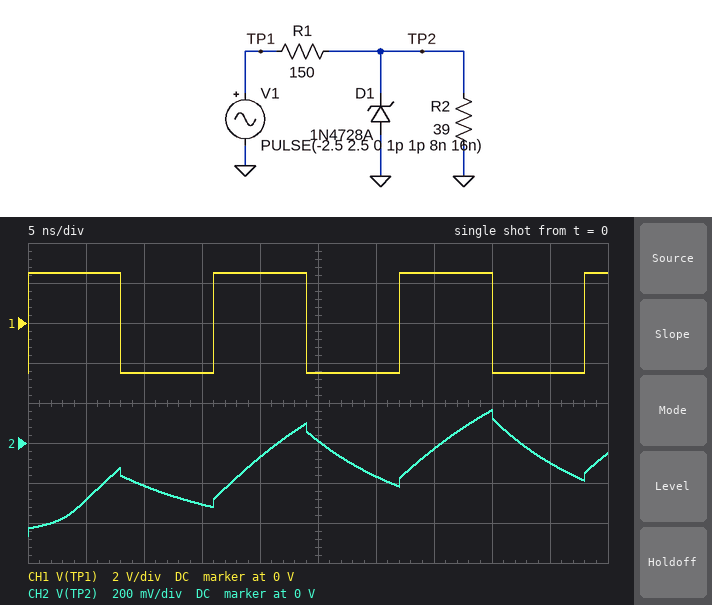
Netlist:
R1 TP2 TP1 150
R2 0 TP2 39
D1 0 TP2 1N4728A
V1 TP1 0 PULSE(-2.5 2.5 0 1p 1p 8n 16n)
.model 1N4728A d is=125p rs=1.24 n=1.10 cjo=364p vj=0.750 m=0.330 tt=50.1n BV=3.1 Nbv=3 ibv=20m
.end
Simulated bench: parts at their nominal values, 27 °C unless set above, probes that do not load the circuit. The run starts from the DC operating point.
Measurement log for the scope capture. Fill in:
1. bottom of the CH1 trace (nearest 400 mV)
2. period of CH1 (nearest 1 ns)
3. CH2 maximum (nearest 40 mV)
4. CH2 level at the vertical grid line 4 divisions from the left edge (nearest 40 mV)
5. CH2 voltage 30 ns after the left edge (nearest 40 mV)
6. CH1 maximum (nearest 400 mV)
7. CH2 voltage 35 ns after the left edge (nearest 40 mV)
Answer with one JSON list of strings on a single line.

["-2.4 V", "16 ns", "160 mV", "-80 mV", "-160 mV", "2.4 V", "-40 mV"]
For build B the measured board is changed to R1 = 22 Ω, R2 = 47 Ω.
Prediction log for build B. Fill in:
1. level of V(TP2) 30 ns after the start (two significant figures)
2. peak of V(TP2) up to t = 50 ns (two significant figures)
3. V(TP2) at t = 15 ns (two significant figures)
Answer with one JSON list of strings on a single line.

["-630 mV", "-300 mV", "-650 mV"]
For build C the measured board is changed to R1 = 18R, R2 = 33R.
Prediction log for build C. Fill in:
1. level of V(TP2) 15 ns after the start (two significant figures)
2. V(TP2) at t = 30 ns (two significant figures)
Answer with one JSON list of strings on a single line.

["-660 mV", "-650 mV"]
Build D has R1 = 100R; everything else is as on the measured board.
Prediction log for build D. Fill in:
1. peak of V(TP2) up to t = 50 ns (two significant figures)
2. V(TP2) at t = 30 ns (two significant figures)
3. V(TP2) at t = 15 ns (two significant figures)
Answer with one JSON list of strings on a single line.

["220 mV", "-300 mV", "-470 mV"]
